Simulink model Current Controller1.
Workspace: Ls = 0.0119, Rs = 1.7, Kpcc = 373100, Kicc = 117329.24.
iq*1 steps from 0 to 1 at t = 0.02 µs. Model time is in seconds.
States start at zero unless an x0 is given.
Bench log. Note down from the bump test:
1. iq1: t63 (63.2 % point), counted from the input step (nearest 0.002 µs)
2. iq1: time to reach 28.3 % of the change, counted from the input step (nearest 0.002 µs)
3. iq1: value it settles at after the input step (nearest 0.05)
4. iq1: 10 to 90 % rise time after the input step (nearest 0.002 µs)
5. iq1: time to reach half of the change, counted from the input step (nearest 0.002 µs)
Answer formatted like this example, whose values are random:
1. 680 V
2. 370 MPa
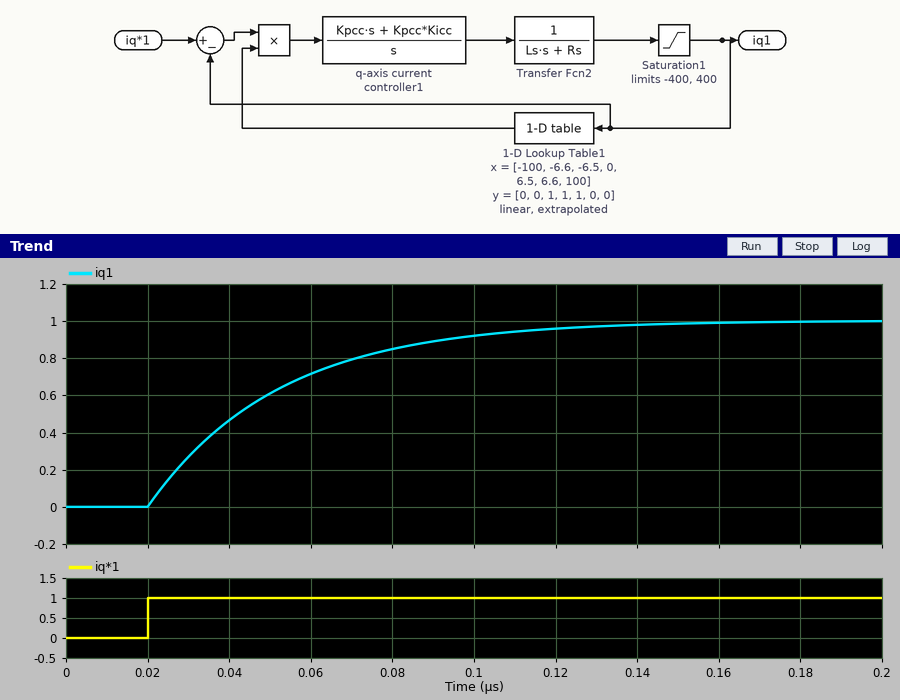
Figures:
1. 0.032 µs
2. 0.010 µs
3. 1.00
4. 0.070 µs
5. 0.022 µs
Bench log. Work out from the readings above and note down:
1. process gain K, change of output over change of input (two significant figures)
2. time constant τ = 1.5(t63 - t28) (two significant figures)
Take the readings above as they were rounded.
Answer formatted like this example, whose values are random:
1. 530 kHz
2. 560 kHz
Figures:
1. 1.0
2. 0.033 µs
